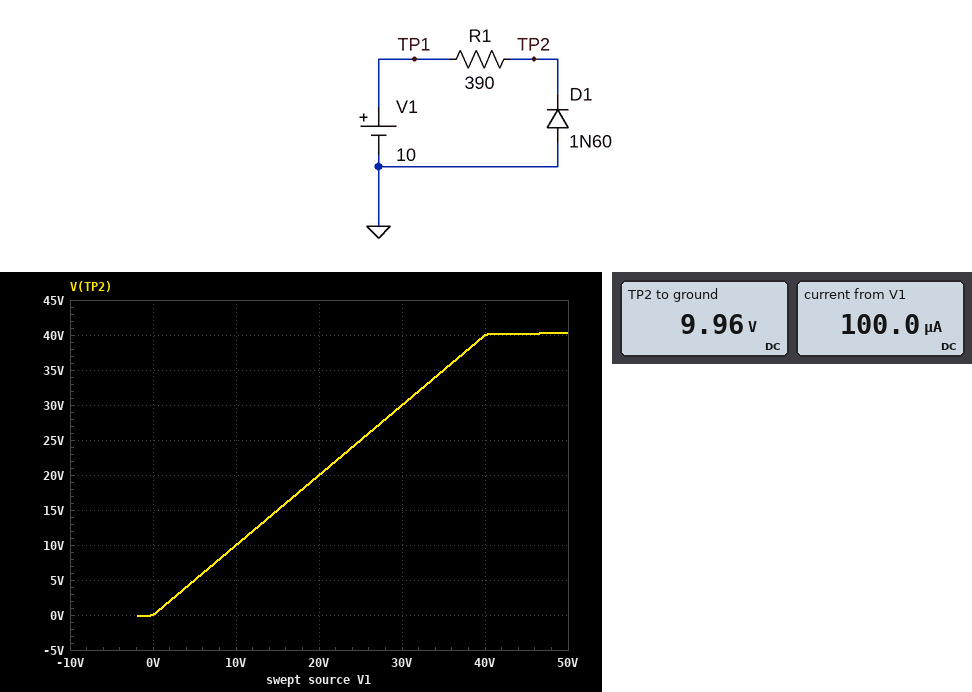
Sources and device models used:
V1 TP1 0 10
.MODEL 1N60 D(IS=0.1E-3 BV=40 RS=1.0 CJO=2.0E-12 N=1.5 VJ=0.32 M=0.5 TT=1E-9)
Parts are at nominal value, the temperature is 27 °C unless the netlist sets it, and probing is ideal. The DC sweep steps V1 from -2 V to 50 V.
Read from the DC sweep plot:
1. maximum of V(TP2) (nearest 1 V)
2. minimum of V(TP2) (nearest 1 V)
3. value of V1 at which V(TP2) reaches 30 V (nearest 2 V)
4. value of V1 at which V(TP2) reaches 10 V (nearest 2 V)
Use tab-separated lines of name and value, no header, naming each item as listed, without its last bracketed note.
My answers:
maximum of V(TP2)	40 V
minimum of V(TP2)	0 V
value of V1 at which V(TP2) reaches 30 V	30 V
value of V1 at which V(TP2) reaches 10 V	10 V
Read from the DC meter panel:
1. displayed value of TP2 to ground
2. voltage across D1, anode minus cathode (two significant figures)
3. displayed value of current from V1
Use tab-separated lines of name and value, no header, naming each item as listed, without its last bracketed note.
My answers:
displayed value of TP2 to ground	9.96 V
voltage across D1, anode minus cathode	-10 V
displayed value of current from V1	100.0 µA
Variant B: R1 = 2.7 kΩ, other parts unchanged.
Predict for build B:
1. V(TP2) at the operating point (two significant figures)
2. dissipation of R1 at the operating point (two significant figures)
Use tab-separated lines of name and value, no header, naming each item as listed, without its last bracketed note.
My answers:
V(TP2) at the operating point	9.7 V
dissipation of R1 at the operating point	27 µW
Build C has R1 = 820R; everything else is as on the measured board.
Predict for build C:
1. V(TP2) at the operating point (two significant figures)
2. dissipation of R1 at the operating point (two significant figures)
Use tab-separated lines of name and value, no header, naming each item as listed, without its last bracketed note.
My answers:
V(TP2) at the operating point	9.9 V
dissipation of R1 at the operating point	8.2 µW
